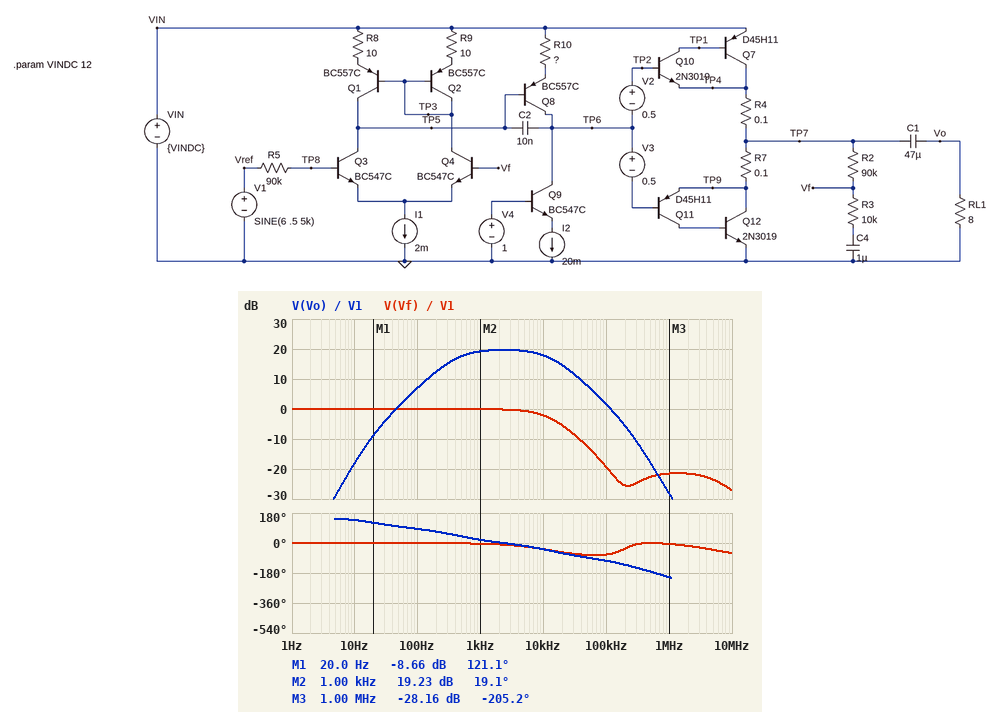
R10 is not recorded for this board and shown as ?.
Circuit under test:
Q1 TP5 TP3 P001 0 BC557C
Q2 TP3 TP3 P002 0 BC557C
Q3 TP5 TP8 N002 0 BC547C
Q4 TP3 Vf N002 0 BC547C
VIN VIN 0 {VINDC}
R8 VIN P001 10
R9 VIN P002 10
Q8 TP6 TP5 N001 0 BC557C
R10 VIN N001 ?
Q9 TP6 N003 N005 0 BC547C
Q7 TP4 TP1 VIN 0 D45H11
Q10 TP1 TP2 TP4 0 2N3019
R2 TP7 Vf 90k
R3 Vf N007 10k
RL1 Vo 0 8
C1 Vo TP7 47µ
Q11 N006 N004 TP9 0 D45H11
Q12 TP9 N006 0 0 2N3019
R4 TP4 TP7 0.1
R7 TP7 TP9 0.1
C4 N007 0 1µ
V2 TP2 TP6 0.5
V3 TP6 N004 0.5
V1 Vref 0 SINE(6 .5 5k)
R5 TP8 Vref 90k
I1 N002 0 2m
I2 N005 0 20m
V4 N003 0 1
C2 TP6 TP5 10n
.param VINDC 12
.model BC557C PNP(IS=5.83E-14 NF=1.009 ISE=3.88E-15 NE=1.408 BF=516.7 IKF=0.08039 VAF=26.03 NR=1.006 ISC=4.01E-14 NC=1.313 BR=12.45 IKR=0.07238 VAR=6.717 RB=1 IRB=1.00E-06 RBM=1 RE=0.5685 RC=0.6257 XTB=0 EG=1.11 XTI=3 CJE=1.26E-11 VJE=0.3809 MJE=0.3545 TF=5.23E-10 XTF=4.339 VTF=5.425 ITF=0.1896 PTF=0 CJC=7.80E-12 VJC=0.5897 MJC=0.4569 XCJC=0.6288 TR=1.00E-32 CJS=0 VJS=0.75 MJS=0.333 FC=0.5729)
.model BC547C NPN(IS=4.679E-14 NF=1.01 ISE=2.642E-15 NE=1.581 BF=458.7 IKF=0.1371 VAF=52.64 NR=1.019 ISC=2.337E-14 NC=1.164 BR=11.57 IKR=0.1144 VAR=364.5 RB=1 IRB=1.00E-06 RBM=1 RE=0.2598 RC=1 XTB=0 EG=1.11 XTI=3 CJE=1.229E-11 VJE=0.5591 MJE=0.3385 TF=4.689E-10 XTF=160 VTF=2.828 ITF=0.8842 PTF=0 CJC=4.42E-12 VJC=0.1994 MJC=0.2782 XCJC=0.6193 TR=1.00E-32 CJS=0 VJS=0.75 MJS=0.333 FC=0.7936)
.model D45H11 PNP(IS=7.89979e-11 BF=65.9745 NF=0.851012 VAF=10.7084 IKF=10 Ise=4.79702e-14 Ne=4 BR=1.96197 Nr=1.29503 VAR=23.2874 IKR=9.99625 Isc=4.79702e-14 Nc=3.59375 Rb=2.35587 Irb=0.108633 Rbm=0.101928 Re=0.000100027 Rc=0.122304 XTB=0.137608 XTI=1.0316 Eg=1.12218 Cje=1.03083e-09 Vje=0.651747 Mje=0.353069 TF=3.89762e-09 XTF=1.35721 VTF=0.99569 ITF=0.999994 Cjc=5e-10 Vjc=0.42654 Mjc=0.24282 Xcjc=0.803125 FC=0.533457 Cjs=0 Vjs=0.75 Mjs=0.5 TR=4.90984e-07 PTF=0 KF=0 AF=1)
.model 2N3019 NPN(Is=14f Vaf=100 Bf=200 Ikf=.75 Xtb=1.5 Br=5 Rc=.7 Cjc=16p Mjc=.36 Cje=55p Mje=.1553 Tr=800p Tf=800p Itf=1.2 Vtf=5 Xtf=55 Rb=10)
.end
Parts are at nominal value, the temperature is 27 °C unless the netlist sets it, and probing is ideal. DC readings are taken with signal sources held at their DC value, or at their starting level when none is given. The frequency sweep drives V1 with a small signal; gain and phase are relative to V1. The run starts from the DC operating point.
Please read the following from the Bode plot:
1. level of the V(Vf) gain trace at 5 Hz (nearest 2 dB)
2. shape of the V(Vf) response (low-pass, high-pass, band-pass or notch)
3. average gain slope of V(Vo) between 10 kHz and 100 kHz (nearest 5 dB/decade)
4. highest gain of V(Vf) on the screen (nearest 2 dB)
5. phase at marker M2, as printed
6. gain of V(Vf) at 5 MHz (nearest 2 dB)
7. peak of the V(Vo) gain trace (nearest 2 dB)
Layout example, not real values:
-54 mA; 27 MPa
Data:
0 dB; low-pass; -15 dB/decade; 0 dB; 19.1 deg; -24 dB; 20 dB
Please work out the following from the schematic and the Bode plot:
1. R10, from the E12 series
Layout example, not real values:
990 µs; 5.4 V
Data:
6.8 Ω
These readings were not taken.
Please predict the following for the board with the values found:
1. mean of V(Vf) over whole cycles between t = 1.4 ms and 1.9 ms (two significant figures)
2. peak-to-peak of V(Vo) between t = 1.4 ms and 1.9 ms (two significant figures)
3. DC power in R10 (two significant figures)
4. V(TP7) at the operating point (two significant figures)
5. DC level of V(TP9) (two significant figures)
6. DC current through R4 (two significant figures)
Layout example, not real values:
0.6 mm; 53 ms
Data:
5.8 V; 9.2 V; 2.7 mW; 6.0 V; 6.0 V; 95 mA
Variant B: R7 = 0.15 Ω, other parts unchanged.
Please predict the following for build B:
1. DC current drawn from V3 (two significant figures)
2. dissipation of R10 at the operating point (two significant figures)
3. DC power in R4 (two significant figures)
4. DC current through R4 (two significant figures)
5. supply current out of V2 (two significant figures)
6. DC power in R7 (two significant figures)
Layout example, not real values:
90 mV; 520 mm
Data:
4.9 µA; 2.7 mW; 790 µW; 89 mA; 4.3 µA; 1.2 mW
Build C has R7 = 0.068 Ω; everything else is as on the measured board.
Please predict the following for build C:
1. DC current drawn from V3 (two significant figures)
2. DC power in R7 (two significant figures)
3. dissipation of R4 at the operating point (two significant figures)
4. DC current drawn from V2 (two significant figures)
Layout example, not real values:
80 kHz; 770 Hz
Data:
5.6 µA; 670 µW; 990 µW; 4.8 µA
